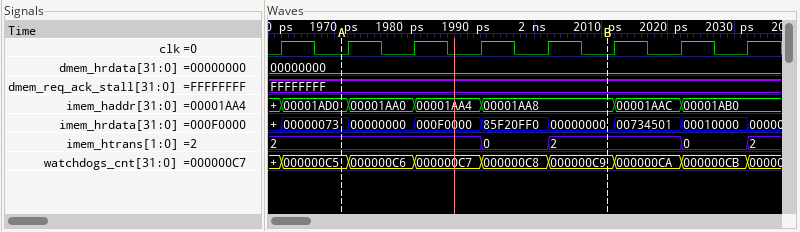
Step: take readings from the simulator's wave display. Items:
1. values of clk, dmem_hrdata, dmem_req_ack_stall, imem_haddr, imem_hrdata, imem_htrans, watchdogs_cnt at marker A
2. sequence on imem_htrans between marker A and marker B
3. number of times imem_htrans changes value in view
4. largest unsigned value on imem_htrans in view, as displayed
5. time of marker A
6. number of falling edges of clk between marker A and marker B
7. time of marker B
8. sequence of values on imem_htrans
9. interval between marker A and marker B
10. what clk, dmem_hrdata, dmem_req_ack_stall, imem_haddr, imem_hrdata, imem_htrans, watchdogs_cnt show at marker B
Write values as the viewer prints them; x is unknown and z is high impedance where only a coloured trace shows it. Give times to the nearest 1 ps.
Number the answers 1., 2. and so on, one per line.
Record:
1. clk=0, dmem_hrdata=00000000, dmem_req_ack_stall=FFFFFFFF, imem_haddr=00001AD0, imem_hrdata=00000073, imem_htrans=2, watchdogs_cnt=000000C5
2. 2, 0, 2
3. 4
4. 2
5. 1971 ps
6. 4
7. 2011 ps
8. 2, 0, 2, 0, 2
9. 40 ps
10. clk=0, dmem_hrdata=00000000, dmem_req_ack_stall=FFFFFFFF, imem_haddr=00001AA8, imem_hrdata=00000000, imem_htrans=2, watchdogs_cnt=000000C9
